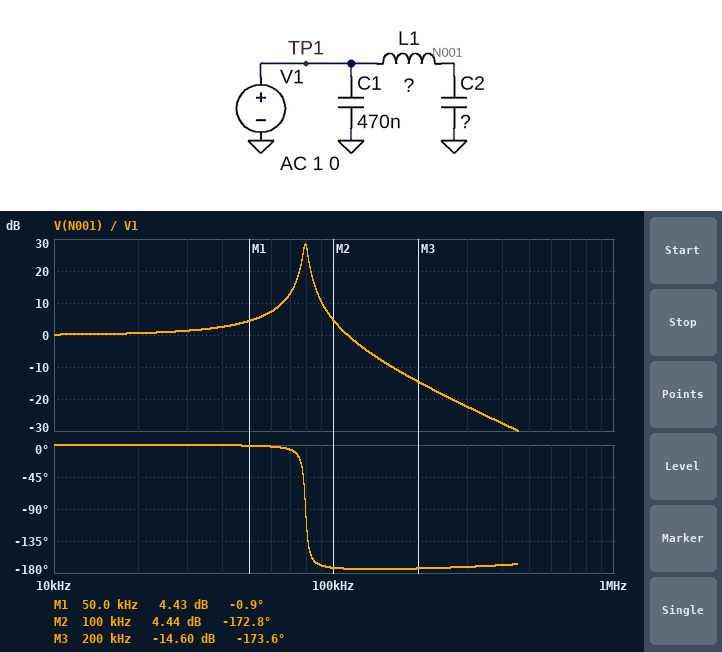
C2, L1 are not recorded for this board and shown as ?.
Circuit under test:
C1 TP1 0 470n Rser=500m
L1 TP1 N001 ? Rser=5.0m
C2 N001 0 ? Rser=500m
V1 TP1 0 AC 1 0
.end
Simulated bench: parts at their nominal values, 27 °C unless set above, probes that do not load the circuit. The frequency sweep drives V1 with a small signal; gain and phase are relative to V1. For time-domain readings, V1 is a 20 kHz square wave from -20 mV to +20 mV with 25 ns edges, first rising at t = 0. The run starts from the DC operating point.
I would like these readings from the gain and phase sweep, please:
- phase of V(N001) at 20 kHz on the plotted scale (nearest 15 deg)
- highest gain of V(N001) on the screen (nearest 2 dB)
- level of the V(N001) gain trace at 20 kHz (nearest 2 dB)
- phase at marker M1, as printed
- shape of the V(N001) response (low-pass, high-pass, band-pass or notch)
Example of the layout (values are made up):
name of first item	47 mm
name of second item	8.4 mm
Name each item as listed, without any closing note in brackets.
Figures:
phase of V(N001) at 20 kHz on the plotted scale	0 deg
highest gain of V(N001) on the screen	28 dB
level of the V(N001) gain trace at 20 kHz	0 dB
phase at marker M1, as printed	-0.9 deg
shape of the V(N001) response	low-pass
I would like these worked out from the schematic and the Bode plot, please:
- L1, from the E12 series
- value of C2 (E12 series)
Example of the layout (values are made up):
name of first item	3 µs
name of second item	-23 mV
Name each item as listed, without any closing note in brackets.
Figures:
L1, from the E12 series	27 µH
value of C2	150 nF
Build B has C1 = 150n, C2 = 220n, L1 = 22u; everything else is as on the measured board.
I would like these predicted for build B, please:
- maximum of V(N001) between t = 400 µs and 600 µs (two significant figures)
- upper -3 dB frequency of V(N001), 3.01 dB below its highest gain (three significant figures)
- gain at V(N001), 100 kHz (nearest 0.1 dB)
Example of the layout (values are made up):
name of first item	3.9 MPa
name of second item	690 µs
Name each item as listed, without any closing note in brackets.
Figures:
maximum of V(N001) between t = 400 µs and 600 µs	46 mV
upper -3 dB frequency of V(N001), 3.01 dB below its highest gain	74.1 kHz
gain at V(N001), 100 kHz	0.8 dB
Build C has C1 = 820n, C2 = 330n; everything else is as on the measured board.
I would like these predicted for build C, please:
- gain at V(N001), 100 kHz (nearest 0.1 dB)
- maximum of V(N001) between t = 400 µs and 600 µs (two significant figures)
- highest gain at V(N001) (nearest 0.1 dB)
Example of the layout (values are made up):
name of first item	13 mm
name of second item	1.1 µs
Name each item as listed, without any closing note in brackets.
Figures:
gain at V(N001), 100 kHz	-8.0 dB
maximum of V(N001) between t = 400 µs and 600 µs	59 mV
highest gain at V(N001)	25.1 dB
